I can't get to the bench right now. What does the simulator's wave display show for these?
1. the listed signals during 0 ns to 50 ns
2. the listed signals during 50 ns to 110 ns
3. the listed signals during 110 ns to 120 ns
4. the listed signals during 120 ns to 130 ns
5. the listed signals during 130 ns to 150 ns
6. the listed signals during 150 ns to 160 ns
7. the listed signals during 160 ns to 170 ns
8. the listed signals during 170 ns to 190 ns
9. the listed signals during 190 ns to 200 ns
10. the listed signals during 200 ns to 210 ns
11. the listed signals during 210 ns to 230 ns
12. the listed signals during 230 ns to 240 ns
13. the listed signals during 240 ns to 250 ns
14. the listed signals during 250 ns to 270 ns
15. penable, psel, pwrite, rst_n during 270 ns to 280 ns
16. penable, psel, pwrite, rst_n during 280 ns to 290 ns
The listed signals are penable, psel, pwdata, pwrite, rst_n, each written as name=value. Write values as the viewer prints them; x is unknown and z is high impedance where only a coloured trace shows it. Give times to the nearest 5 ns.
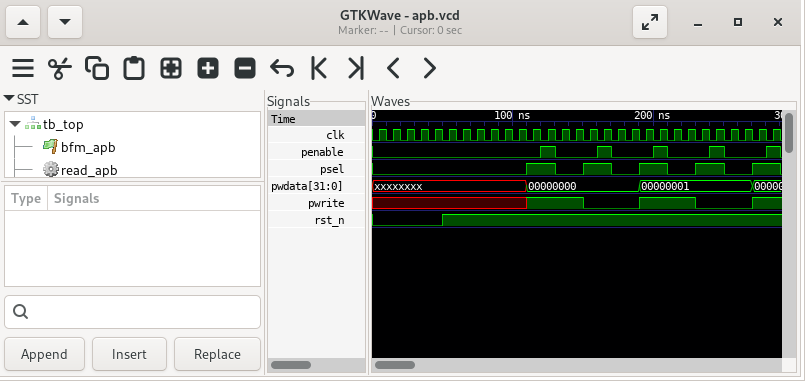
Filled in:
penable=0, psel=0, pwdata=xxxxxxxx, pwrite=x, rst_n=0
penable=0, psel=0, pwdata=xxxxxxxx, pwrite=x, rst_n=1
penable=0, psel=1, pwdata=00000000, pwrite=1, rst_n=1
penable=1, psel=1, pwdata=00000000, pwrite=1, rst_n=1
penable=0, psel=0, pwdata=00000000, pwrite=1, rst_n=1
penable=0, psel=1, pwdata=00000000, pwrite=0, rst_n=1
penable=1, psel=1, pwdata=00000000, pwrite=0, rst_n=1
penable=0, psel=0, pwdata=00000000, pwrite=0, rst_n=1
penable=0, psel=1, pwdata=00000001, pwrite=1, rst_n=1
penable=1, psel=1, pwdata=00000001, pwrite=1, rst_n=1
penable=0, psel=0, pwdata=00000001, pwrite=1, rst_n=1
penable=0, psel=1, pwdata=00000001, pwrite=0, rst_n=1
penable=1, psel=1, pwdata=00000001, pwrite=0, rst_n=1
penable=0, psel=0, pwdata=00000001, pwrite=0, rst_n=1
penable=0, psel=1, pwrite=1, rst_n=1
penable=1, psel=1, pwrite=1, rst_n=1
